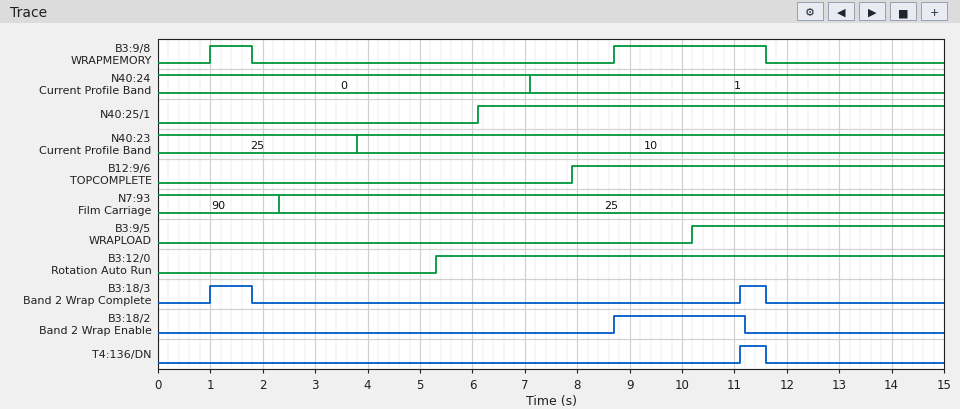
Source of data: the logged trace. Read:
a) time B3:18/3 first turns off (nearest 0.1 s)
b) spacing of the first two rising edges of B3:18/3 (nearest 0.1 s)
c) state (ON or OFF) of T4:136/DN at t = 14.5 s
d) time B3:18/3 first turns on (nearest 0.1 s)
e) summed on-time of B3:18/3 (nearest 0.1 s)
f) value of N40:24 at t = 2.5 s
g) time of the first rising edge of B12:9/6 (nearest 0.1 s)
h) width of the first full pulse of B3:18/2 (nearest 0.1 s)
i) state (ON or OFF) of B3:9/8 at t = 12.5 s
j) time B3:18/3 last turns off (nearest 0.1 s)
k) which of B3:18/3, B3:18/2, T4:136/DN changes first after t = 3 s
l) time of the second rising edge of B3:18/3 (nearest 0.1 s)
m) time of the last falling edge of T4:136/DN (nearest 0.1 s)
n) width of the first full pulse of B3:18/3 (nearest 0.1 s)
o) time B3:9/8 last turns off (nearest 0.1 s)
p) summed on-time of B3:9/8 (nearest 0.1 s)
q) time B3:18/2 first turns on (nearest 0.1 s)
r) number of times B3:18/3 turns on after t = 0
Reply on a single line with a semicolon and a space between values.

1.8 s; 10.1 s; OFF; 1.0 s; 1.3 s; 0; 7.9 s; 2.5 s; OFF; 11.6 s; B3:18/2; 11.1 s; 11.6 s; 0.8 s; 11.6 s; 3.7 s; 8.7 s; 2
